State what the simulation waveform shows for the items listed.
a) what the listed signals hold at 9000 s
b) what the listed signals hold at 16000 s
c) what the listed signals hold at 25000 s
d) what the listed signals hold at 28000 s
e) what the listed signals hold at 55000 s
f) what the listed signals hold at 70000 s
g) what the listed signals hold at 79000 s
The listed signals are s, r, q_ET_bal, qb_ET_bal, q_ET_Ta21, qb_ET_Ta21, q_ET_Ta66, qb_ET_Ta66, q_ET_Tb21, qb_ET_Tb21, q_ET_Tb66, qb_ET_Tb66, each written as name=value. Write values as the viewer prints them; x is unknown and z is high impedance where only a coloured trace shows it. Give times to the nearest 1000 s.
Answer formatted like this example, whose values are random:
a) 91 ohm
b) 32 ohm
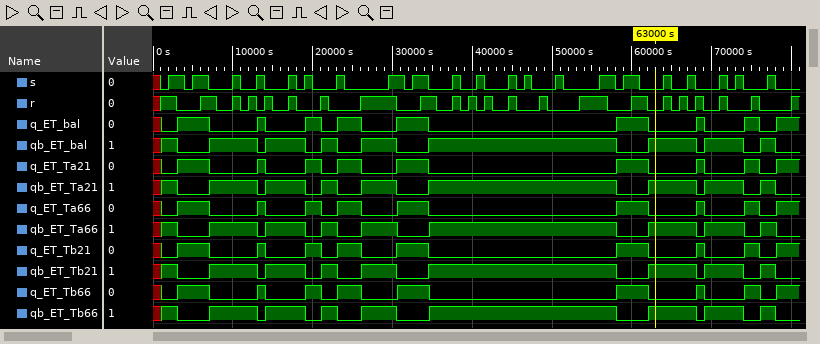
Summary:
a) s=0, r=0, q_ET_bal=0, qb_ET_bal=1, q_ET_Ta21=0, qb_ET_Ta21=1, q_ET_Ta66=0, qb_ET_Ta66=1, q_ET_Tb21=0, qb_ET_Tb21=1, q_ET_Tb66=0, qb_ET_Tb66=1
b) s=0, r=0, q_ET_bal=0, qb_ET_bal=1, q_ET_Ta21=0, qb_ET_Ta21=1, q_ET_Ta66=0, qb_ET_Ta66=1, q_ET_Tb21=0, qb_ET_Tb21=1, q_ET_Tb66=0, qb_ET_Tb66=1
c) s=0, r=0, q_ET_bal=1, qb_ET_bal=0, q_ET_Ta21=1, qb_ET_Ta21=0, q_ET_Ta66=1, qb_ET_Ta66=0, q_ET_Tb21=1, qb_ET_Tb21=0, q_ET_Tb66=1, qb_ET_Tb66=0
d) s=0, r=1, q_ET_bal=0, qb_ET_bal=1, q_ET_Ta21=0, qb_ET_Ta21=1, q_ET_Ta66=0, qb_ET_Ta66=1, q_ET_Tb21=0, qb_ET_Tb21=1, q_ET_Tb66=0, qb_ET_Tb66=1
e) s=0, r=1, q_ET_bal=0, qb_ET_bal=1, q_ET_Ta21=0, qb_ET_Ta21=1, q_ET_Ta66=0, qb_ET_Ta66=1, q_ET_Tb21=0, qb_ET_Tb21=1, q_ET_Tb66=0, qb_ET_Tb66=1
f) s=0, r=0, q_ET_bal=0, qb_ET_bal=1, q_ET_Ta21=0, qb_ET_Ta21=1, q_ET_Ta66=0, qb_ET_Ta66=1, q_ET_Tb21=0, qb_ET_Tb21=1, q_ET_Tb66=0, qb_ET_Tb66=1
g) s=0, r=0, q_ET_bal=1, qb_ET_bal=0, q_ET_Ta21=1, qb_ET_Ta21=0, q_ET_Ta66=1, qb_ET_Ta66=0, q_ET_Tb21=1, qb_ET_Tb21=0, q_ET_Tb66=1, qb_ET_Tb66=0
